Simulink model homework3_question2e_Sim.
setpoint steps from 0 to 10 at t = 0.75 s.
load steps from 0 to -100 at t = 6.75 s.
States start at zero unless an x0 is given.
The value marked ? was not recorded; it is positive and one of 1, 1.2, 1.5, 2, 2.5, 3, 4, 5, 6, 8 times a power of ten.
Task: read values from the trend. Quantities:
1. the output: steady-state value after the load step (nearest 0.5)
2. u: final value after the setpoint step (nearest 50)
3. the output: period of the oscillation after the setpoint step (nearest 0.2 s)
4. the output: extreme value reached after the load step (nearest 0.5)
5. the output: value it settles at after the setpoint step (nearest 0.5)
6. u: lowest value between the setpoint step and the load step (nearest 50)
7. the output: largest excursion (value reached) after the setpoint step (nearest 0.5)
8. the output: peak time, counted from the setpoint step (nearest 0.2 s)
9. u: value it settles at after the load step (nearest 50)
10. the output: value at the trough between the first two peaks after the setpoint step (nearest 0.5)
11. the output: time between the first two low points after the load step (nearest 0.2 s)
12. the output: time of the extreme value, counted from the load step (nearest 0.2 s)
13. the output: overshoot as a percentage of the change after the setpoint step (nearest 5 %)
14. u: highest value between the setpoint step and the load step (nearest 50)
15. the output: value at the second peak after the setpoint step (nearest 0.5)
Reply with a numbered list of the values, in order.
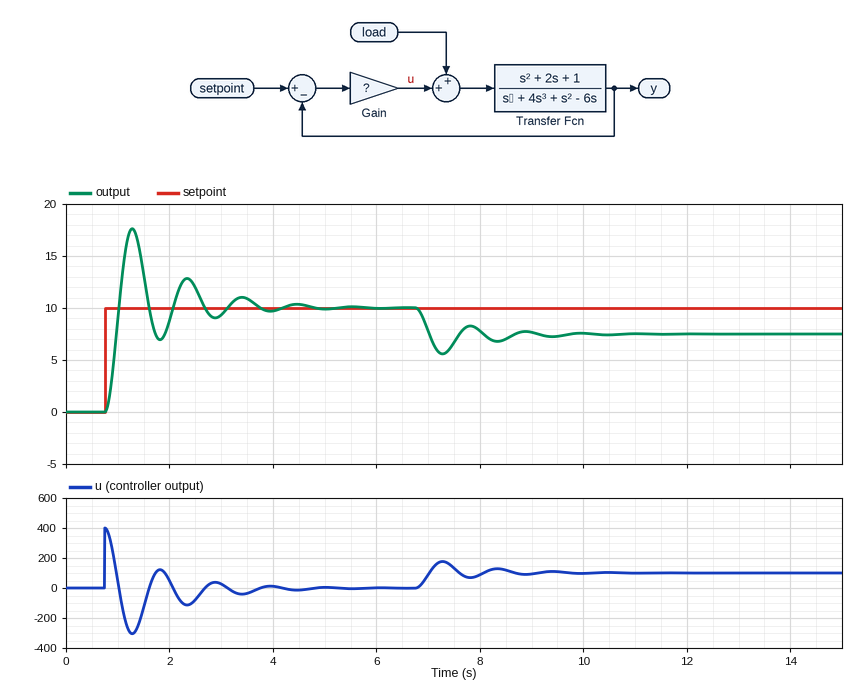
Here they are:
1. 7.5
2. 0
3. 1.0 s
4. 5.5
5. 10.0
6. -300
7. 17.5
8. 0.6 s
9. 100
10. 7.0
11. 1.0 s
12. 0.6 s
13. 75 %
14. 400
15. 13.0
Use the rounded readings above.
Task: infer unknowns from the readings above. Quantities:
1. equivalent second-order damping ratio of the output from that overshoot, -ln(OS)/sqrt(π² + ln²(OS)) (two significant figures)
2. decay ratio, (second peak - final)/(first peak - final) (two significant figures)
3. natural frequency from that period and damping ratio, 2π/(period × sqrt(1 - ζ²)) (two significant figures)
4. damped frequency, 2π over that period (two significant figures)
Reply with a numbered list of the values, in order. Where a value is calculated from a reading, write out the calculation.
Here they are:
1. ln(0.75) = -0.288; 0.288 / sqrt(9.870 + 0.083) = 0.091
2. (13 - 10) / (17.5 - 10) = 0.40
3. 2π / (1 × sqrt(1 - 0.091²)) = 6.3 rad/s
4. 2π / 1 = 6.3 rad/s
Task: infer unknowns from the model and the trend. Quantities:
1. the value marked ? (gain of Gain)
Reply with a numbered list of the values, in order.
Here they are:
1. 40
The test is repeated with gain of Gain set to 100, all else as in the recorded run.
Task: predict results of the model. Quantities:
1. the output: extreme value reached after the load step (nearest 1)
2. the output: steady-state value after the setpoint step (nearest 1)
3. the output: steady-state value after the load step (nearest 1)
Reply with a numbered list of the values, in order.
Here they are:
1. 8
2. 10
3. 9
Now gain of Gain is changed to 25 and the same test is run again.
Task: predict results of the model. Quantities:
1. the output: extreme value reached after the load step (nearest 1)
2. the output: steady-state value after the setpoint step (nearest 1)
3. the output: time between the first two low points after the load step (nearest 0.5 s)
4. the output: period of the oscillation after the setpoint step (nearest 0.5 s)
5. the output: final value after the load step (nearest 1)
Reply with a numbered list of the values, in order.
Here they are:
1. 3
2. 10
3. 1.5 s
4. 1.5 s
5. 6
